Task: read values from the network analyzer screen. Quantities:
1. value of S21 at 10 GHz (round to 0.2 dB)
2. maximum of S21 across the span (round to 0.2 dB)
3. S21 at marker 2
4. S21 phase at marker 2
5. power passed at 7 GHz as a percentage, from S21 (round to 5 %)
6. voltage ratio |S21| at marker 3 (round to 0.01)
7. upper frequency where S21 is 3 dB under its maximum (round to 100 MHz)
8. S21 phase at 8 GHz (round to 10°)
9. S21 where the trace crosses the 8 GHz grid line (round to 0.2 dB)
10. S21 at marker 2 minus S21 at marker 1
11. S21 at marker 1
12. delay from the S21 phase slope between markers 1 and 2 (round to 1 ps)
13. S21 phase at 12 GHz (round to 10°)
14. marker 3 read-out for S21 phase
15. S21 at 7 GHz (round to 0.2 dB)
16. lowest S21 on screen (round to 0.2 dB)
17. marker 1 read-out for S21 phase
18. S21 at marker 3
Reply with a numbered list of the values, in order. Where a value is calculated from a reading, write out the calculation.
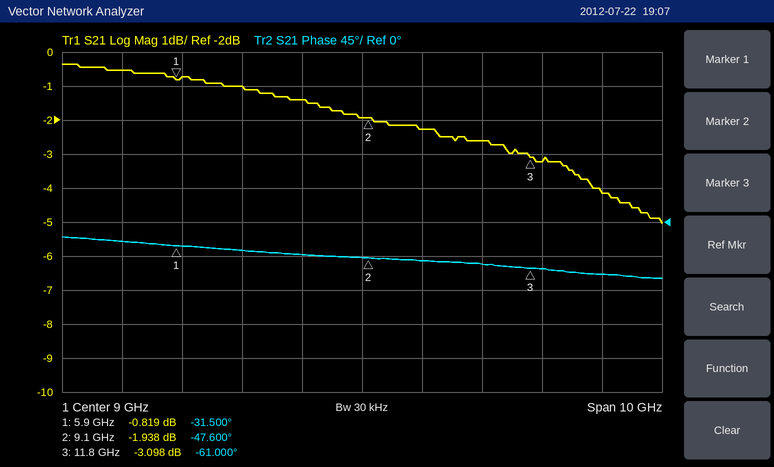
1. -2.2 dB
2. -0.4 dB
3. -1.938 dB
4. -47.600°
5. 10^(-1/10) ≈ 79.4 %, so 80 % to the nearest 5 %
6. 10^(-3.098/20) ≈ 0.70
7. 12.4 GHz
8. -40°
9. -1.4 dB
10. -1.938 − (-0.819) = -1.119 dB
11. -0.819 dB
12. −(-47.6° − (-31.5°))/(360° × 3.2 GHz) ≈ 14 ps
13. -60°
14. -61.000°
15. -1.0 dB
16. -5.0 dB
17. -31.500°
18. -3.098 dB
